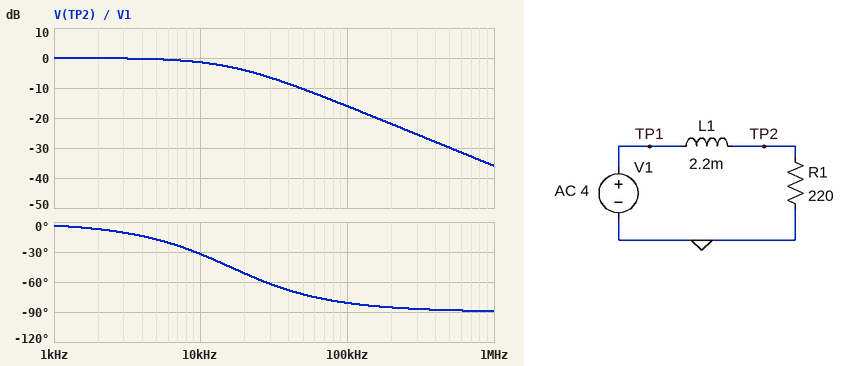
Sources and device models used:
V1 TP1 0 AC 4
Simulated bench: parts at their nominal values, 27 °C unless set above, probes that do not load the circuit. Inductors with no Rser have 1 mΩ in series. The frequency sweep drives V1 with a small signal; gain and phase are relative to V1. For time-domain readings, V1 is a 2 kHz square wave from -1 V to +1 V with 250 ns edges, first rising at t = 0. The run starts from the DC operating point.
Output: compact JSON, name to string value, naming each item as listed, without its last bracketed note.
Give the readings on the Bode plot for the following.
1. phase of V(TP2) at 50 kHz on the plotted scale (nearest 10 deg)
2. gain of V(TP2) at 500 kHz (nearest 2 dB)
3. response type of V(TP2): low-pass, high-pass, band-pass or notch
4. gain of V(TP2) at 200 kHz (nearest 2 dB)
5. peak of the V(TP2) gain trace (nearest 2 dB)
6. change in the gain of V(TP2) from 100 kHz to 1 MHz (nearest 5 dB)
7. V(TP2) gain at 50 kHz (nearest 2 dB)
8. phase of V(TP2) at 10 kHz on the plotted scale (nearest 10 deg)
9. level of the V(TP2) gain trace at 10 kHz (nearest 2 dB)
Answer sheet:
{"phase of V(TP2) at 50 kHz on the plotted scale": "-70 deg", "gain of V(TP2) at 500 kHz": "-30 dB", "response type of V(TP2): low-pass, high-pass, band-pass or notch": "low-pass", "gain of V(TP2) at 200 kHz": "-22 dB", "peak of the V(TP2) gain trace": "0 dB", "change in the gain of V(TP2) from 100 kHz to 1 MHz": "-20 dB", "V(TP2) gain at 50 kHz": "-10 dB", "phase of V(TP2) at 10 kHz on the plotted scale": "-30 deg", "level of the V(TP2) gain trace at 10 kHz": "-2 dB"}
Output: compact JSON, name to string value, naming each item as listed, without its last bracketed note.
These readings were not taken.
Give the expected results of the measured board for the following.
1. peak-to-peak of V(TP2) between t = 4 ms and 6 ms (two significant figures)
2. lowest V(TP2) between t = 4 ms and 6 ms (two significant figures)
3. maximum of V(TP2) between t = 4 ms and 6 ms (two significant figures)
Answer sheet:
{"peak-to-peak of V(TP2) between t = 4 ms and 6 ms": "2.0 V", "lowest V(TP2) between t = 4 ms and 6 ms": "-1.0 V", "maximum of V(TP2) between t = 4 ms and 6 ms": "1.0 V"}
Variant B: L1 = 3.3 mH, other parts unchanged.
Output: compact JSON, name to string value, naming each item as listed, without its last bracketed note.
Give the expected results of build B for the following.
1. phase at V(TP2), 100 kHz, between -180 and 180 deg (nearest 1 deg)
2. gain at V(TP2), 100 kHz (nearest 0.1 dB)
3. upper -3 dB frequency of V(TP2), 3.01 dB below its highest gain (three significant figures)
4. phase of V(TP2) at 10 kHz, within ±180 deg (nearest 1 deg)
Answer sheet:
{"phase at V(TP2), 100 kHz, between -180 and 180 deg": "-84 deg", "gain at V(TP2), 100 kHz": "-19.5 dB", "upper -3 dB frequency of V(TP2), 3.01 dB below its highest gain": "10.6 kHz", "phase of V(TP2) at 10 kHz, within ±180 deg": "-43 deg"}
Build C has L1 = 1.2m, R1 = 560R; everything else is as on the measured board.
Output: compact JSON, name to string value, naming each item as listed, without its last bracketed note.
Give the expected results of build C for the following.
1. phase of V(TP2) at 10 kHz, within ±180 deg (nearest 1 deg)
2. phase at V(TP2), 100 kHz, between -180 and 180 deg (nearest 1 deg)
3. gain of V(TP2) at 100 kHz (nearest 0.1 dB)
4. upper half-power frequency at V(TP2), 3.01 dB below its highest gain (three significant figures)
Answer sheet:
{"phase of V(TP2) at 10 kHz, within ±180 deg": "-8 deg", "phase at V(TP2), 100 kHz, between -180 and 180 deg": "-53 deg", "gain of V(TP2) at 100 kHz": "-4.5 dB", "upper half-power frequency at V(TP2), 3.01 dB below its highest gain": "74.3 kHz"}
